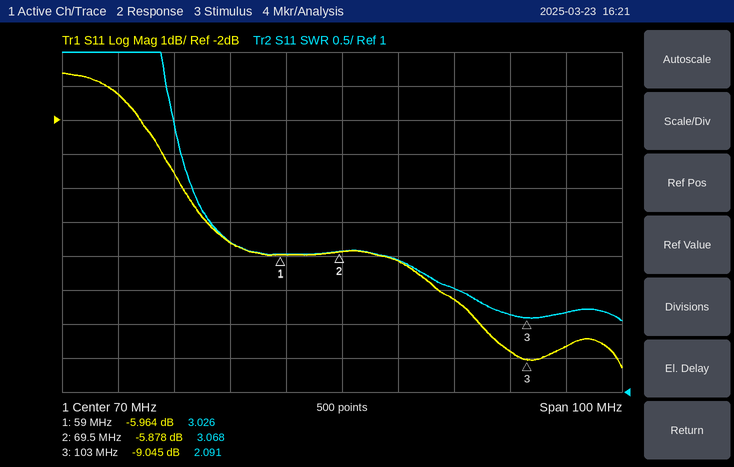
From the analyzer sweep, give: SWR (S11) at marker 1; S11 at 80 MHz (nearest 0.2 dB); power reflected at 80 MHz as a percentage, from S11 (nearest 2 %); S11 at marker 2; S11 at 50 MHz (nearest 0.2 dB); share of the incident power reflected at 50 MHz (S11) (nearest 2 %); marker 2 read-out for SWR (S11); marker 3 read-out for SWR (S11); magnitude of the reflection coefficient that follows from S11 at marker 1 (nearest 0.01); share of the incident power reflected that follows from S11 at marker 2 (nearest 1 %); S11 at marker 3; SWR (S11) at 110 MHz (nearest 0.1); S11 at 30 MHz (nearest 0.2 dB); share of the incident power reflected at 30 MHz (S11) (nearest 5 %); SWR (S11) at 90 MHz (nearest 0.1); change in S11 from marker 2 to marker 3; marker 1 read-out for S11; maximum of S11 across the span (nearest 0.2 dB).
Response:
3.026
-6.2 dB
24 %
-5.878 dB
-5.6 dB
28 %
3.068
2.091
0.50
26 %
-9.045 dB
2.2
-1.2 dB
75 %
2.5
-3.167 dB
-5.964 dB
-0.6 dB
